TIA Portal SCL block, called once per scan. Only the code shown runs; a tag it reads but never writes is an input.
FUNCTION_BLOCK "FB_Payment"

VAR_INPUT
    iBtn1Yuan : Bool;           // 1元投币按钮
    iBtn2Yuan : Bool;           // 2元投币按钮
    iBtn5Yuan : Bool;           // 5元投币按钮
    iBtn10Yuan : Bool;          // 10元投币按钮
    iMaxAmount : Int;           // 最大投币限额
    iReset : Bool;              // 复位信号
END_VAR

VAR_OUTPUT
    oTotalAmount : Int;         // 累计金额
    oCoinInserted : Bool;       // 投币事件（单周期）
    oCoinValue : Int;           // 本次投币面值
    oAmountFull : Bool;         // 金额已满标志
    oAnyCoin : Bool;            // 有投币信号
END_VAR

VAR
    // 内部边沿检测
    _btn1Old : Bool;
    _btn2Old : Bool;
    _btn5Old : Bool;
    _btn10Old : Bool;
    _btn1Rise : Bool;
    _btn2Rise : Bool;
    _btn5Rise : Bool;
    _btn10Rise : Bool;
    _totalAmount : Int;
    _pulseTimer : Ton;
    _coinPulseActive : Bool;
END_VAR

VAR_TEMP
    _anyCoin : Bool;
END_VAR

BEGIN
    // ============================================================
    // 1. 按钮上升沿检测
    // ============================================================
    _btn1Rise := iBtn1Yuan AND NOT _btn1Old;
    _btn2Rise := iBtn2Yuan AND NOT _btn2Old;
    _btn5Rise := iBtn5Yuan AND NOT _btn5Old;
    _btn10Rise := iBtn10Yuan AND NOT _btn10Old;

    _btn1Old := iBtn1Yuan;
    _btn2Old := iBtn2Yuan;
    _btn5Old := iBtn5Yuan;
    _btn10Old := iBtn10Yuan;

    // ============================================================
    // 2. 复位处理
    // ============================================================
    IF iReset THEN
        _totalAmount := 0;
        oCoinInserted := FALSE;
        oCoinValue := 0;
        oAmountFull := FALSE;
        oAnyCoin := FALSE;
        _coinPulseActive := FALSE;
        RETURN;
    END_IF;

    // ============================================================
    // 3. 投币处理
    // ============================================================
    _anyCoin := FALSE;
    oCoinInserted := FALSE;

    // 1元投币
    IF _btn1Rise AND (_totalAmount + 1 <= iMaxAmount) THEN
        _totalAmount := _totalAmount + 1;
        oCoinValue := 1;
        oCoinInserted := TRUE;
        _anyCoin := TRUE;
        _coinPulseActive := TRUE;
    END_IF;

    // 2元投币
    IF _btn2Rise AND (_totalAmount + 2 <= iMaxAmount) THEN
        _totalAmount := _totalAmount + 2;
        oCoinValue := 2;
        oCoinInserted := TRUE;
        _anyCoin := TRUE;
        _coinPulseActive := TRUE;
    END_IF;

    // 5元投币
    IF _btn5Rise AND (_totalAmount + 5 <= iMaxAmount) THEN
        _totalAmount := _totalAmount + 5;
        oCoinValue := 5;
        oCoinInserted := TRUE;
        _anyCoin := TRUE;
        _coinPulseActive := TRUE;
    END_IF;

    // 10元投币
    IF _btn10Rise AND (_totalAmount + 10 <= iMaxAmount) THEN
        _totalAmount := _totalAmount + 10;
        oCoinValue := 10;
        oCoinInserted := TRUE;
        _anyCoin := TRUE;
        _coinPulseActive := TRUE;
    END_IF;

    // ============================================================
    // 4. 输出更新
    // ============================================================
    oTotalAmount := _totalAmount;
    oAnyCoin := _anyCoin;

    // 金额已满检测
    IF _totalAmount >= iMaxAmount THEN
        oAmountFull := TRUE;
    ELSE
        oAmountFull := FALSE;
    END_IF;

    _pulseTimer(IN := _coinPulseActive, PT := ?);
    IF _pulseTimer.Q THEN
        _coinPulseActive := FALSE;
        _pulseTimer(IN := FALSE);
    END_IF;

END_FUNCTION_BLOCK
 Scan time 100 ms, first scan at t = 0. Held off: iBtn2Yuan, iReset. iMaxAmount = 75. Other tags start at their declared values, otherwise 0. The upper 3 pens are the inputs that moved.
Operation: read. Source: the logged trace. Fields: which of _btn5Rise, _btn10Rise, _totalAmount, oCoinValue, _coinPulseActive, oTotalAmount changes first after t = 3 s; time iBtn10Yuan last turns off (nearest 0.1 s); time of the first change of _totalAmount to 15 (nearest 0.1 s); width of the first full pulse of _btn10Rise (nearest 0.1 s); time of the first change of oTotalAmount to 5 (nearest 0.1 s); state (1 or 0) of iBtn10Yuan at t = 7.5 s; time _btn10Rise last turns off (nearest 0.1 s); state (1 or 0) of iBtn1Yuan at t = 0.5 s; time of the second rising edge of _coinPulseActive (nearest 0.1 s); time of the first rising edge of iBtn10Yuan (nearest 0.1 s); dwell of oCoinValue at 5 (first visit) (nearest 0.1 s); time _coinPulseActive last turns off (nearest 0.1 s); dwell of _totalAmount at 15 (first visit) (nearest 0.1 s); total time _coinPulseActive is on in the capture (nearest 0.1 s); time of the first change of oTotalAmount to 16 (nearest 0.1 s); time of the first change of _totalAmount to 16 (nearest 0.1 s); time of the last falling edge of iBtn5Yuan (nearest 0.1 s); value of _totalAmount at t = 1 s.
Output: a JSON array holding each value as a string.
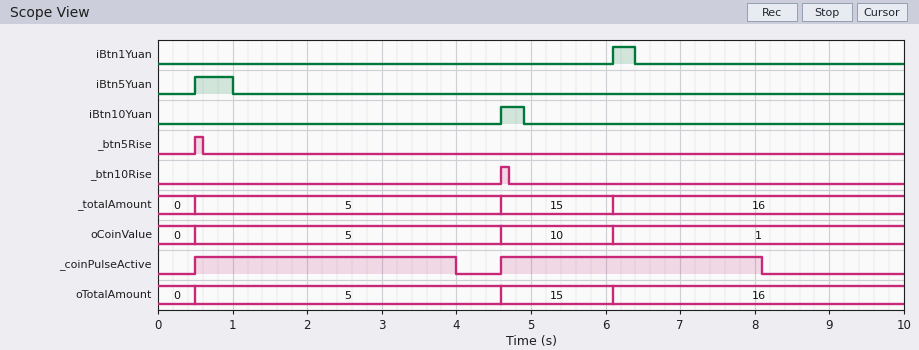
["_coinPulseActive", "4.9 s", "4.6 s", "0.1 s", "0.5 s", "0", "4.7 s", "0", "4.6 s", "4.6 s", "4.1 s", "8.1 s", "1.5 s", "7.0 s", "6.1 s", "6.1 s", "1.0 s", "5"]
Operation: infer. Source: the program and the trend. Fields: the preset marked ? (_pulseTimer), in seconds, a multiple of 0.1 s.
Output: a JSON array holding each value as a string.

["3.5 s"]
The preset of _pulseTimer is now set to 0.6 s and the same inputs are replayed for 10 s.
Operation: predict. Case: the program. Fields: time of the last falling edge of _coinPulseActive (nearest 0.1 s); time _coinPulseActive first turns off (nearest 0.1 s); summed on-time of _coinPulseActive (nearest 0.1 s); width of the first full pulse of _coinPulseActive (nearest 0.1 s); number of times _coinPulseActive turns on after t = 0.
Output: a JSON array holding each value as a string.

["6.7 s", "1.1 s", "1.8 s", "0.6 s", "3"]
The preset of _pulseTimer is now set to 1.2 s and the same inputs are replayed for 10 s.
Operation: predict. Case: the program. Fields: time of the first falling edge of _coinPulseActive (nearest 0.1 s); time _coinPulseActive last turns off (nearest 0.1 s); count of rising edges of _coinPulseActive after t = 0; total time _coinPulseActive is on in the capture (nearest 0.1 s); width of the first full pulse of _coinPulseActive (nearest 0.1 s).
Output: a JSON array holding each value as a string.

["1.7 s", "7.3 s", "3", "3.6 s", "1.2 s"]
